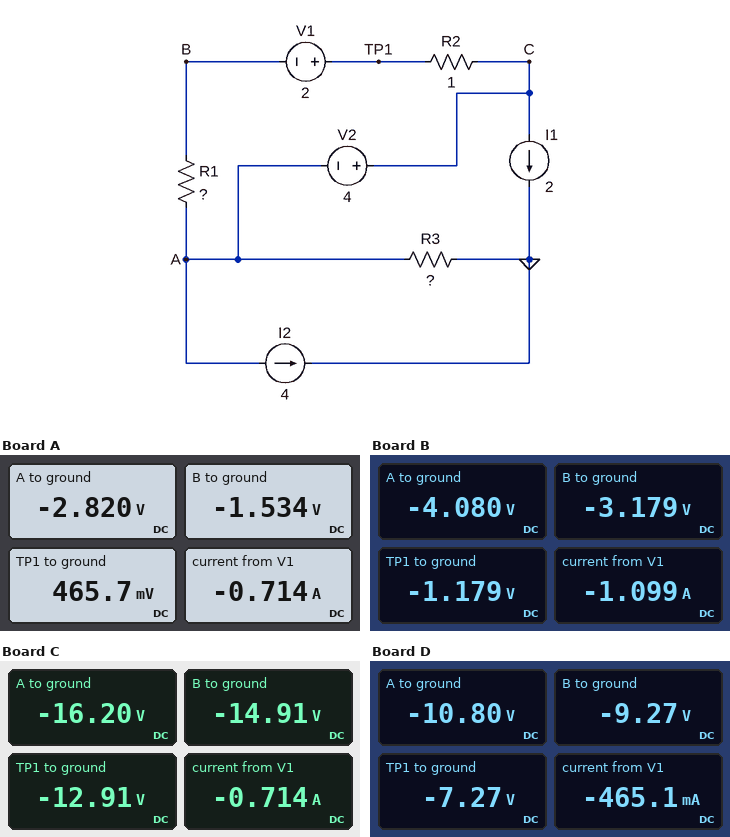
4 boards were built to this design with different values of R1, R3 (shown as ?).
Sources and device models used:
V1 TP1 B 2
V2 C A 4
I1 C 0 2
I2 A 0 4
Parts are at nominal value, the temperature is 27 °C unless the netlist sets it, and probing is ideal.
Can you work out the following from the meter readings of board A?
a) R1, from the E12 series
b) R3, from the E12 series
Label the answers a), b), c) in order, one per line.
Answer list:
a) 1.8 Ω
b) 0.47 Ω
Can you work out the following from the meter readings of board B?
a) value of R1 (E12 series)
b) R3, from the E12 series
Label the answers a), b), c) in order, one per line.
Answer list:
a) 0.82 Ω
b) 0.68 Ω
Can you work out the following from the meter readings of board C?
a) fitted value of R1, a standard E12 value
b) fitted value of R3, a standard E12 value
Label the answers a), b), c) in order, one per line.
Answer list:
a) 1.8 Ω
b) 2.7 Ω
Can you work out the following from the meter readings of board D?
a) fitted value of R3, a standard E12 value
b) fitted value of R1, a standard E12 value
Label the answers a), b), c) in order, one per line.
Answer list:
a) 1.8 Ω
b) 3.3 Ω
